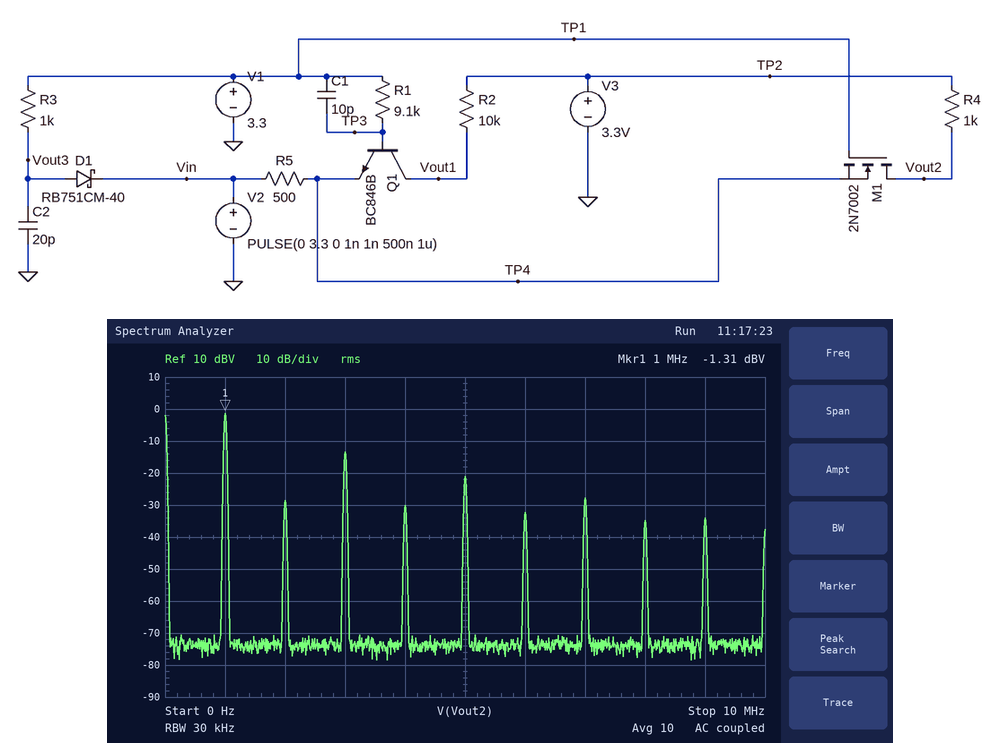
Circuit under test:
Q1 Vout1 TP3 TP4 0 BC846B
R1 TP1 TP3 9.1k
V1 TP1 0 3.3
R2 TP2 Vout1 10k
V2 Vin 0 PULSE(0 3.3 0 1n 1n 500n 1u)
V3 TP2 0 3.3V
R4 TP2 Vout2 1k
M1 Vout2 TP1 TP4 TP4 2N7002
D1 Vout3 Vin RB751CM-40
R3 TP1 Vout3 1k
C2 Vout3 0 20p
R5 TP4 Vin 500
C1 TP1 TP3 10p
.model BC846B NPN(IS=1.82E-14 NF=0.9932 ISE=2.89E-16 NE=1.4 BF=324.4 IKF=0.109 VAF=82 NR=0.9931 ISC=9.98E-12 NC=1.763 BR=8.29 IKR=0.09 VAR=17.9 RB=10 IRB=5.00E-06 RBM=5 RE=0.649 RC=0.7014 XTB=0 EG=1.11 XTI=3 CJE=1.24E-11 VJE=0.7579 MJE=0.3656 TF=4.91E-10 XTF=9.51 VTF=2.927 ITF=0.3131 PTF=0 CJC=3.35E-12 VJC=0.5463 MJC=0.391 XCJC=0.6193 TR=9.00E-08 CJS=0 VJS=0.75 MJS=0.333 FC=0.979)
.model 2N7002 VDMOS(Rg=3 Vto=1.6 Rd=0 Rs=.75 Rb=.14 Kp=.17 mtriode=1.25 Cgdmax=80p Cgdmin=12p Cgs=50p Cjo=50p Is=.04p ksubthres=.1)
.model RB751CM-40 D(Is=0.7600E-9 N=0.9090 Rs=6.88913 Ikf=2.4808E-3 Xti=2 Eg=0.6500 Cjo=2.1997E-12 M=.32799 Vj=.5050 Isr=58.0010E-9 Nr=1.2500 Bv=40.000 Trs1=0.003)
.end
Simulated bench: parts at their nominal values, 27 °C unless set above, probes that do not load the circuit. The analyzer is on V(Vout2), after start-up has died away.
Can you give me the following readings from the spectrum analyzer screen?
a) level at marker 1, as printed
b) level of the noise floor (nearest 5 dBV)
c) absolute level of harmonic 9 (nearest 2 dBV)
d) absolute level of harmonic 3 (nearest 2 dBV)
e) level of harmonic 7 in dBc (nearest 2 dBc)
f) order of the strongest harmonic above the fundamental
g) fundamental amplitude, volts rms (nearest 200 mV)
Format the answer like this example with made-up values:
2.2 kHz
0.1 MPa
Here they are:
-1.31 dBV
-75 dBV
-34 dBV
-14 dBV
-26 dBc
3
800 mV
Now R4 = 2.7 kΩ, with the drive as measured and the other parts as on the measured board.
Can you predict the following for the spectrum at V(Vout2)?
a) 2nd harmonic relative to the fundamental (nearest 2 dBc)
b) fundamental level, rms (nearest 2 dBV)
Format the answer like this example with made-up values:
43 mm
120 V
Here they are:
-24 dBc
0 dBV
